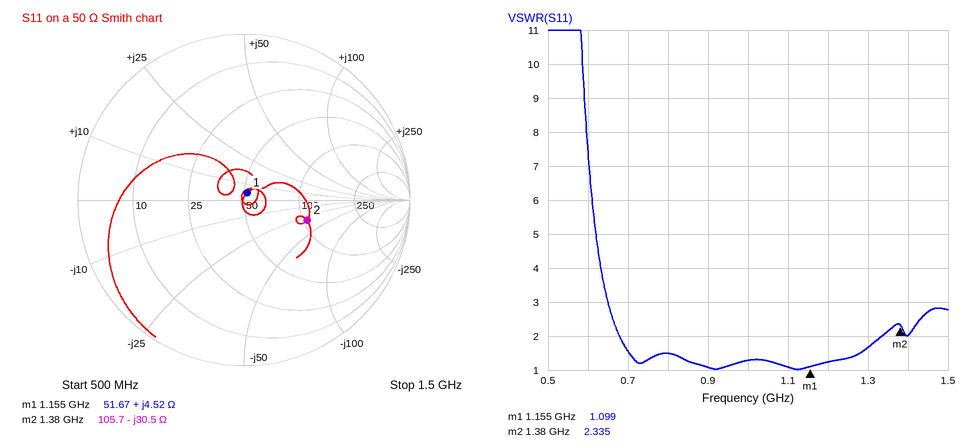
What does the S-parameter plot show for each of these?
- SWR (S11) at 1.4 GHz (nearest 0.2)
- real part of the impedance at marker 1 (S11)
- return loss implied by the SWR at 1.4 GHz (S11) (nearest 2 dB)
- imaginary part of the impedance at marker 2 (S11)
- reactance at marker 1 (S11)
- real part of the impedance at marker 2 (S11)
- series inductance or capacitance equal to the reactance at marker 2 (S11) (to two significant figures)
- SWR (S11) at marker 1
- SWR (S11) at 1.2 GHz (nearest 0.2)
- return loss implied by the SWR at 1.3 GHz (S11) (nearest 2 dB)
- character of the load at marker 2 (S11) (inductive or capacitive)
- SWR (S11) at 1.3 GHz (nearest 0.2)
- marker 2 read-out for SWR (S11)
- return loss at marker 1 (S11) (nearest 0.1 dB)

2.0
51.67 Ω
10 dB
-30.5 Ω
+4.52 Ω
105.7 Ω
3.8 pF
1.099
1.2
12 dB
capacitive
1.6
2.335
26.5 dB
